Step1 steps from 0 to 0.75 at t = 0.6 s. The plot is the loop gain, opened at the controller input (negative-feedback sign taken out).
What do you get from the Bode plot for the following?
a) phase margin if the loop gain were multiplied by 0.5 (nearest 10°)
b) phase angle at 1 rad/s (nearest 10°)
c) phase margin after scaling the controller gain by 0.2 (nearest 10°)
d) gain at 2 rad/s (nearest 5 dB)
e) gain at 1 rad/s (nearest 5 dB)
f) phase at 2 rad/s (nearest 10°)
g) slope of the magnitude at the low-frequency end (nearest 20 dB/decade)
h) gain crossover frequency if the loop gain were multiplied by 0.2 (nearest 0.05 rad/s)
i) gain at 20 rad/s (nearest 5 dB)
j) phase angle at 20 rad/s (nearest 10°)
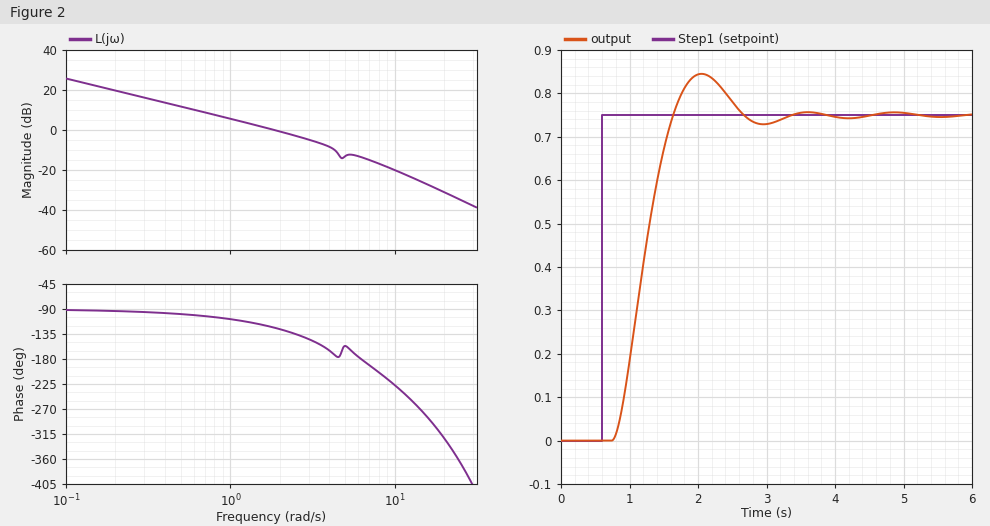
70°
-110°
80°
0 dB
5 dB
-130°
-20 dB/decade
0.40 rad/s
-30 dB
-320°
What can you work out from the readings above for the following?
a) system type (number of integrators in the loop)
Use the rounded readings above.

1
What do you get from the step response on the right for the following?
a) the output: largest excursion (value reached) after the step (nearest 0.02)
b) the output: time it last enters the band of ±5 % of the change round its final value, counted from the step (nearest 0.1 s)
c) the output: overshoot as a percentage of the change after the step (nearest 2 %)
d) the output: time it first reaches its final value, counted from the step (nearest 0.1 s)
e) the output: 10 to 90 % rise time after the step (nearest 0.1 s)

0.84
1.9 s
12 %
1.0 s
0.6 s
